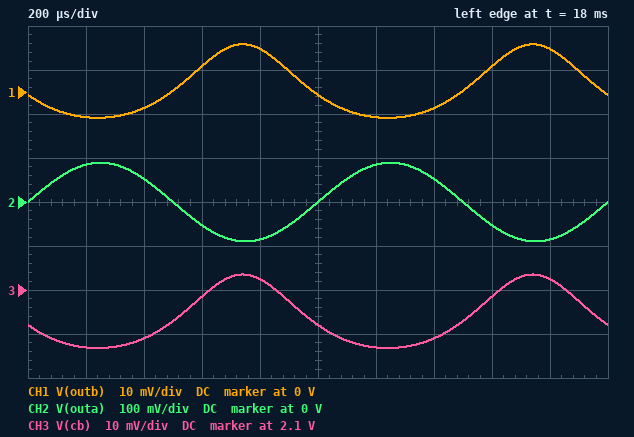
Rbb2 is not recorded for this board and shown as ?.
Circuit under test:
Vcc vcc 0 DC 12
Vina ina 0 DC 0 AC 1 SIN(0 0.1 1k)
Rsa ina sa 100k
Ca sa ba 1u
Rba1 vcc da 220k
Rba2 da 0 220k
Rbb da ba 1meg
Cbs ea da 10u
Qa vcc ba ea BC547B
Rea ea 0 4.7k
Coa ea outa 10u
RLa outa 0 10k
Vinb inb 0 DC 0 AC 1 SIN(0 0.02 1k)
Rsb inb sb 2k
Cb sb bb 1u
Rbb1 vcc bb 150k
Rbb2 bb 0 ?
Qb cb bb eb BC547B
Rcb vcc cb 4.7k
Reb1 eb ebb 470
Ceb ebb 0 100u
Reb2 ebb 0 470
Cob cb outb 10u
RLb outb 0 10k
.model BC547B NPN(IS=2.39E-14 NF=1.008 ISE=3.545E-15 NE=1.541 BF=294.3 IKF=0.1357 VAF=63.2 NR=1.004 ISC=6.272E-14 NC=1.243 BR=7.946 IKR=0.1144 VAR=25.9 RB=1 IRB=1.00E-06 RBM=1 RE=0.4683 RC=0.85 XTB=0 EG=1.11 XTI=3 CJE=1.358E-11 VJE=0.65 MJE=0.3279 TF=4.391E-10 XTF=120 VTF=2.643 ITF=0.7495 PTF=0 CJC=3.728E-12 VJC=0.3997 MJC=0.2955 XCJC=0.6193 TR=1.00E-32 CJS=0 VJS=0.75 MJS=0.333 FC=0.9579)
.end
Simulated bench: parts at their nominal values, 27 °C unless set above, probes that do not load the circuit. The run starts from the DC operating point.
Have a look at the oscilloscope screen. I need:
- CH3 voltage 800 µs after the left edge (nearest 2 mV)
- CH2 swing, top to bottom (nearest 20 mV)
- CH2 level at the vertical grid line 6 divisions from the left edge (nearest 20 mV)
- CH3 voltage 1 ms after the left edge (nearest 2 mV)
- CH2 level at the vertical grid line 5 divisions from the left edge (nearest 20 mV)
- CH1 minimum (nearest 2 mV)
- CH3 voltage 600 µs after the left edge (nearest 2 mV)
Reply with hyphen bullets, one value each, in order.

- 2.102 V
- 180 mV
- 80 mV
- 2.092 V
- 0 V
- -6 mV
- 2.098 V
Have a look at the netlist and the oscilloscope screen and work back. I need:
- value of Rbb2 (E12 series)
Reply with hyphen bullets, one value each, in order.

- 68 kΩ
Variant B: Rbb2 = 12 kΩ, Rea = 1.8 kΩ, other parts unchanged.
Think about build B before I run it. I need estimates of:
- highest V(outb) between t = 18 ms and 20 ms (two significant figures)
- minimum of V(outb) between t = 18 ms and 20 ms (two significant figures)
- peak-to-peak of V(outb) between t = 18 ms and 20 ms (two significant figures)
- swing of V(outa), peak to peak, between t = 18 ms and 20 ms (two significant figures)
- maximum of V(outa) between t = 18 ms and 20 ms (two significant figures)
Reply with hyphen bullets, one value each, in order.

- 95 mV
- -96 mV
- 190 mV
- 160 mV
- 81 mV
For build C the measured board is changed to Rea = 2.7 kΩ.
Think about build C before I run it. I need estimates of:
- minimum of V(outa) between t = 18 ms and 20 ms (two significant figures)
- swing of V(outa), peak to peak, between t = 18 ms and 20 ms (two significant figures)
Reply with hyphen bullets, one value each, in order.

- -86 mV
- 170 mV
